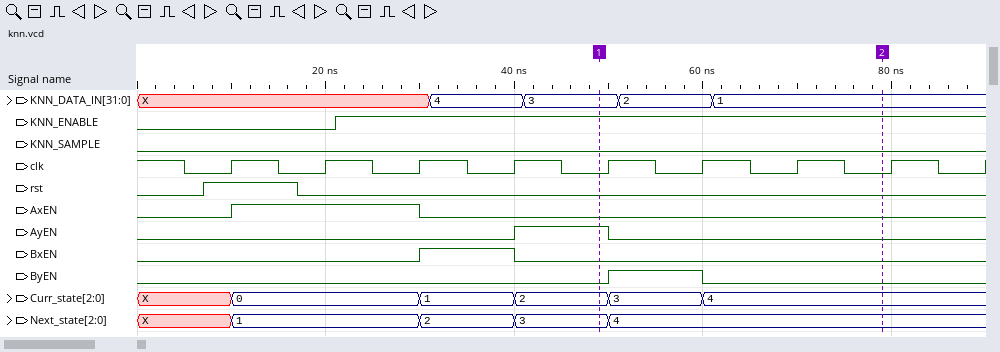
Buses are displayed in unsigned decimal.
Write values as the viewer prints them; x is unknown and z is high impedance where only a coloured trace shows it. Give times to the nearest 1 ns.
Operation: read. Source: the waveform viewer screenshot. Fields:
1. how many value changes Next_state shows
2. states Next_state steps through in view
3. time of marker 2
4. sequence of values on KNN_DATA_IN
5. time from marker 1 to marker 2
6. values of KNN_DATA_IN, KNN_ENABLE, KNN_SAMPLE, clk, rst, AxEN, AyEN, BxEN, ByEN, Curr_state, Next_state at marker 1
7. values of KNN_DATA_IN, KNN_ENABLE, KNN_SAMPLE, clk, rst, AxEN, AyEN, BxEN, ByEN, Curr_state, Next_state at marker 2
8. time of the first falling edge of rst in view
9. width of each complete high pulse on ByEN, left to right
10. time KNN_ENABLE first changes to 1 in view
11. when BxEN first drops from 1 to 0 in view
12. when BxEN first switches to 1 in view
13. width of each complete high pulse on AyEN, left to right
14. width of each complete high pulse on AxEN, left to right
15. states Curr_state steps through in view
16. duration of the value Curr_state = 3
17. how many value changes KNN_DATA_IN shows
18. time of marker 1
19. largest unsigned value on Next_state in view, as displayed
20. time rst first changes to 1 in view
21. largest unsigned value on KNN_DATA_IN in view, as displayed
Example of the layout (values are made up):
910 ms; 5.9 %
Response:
4; X, 1, 2, 3, 4; 79 ns; X, 4, 3, 2, 1; 30 ns; KNN_DATA_IN=3, KNN_ENABLE=1, KNN_SAMPLE=0, clk=0, rst=0, AxEN=0, AyEN=1, BxEN=0, ByEN=0, Curr_state=2, Next_state=3; KNN_DATA_IN=1, KNN_ENABLE=1, KNN_SAMPLE=0, clk=0, rst=0, AxEN=0, AyEN=0, BxEN=0, ByEN=0, Curr_state=4, Next_state=4; 17 ns; 10 ns; 21 ns; 40 ns; 30 ns; 10 ns; 20 ns; X, 0, 1, 2, 3, 4; 10 ns; 4; 49 ns; 4; 7 ns; 4
